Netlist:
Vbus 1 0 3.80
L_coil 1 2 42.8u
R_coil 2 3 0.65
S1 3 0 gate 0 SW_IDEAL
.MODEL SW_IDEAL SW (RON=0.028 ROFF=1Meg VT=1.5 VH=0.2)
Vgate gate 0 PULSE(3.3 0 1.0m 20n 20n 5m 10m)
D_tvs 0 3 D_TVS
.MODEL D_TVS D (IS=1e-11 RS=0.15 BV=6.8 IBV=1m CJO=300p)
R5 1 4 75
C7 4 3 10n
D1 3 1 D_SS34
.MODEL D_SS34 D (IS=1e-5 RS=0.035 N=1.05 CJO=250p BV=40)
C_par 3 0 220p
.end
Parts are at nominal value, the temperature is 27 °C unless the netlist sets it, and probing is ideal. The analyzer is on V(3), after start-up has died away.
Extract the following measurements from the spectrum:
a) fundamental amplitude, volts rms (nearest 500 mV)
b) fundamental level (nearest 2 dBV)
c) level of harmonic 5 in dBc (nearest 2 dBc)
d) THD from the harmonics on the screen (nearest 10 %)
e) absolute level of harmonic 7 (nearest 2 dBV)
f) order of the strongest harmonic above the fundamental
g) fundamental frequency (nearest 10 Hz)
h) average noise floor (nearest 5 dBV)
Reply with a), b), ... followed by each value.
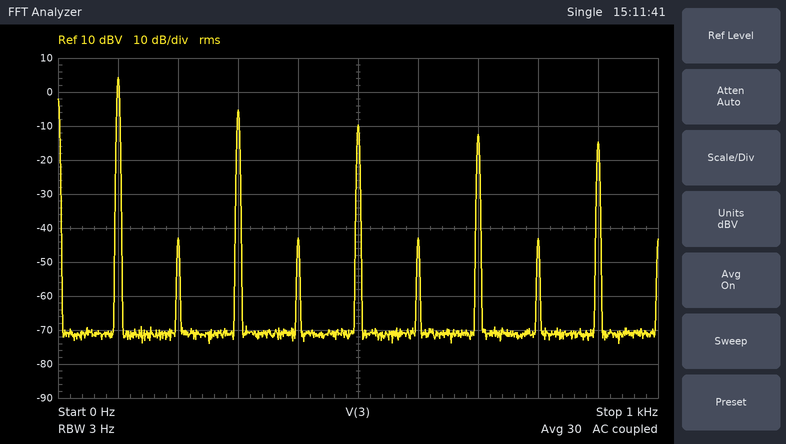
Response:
a) 1.5 V
b) 4 dBV
c) -14 dBc
d) 40 %
e) -12 dBV
f) 3
g) 100 Hz
h) -70 dBV
